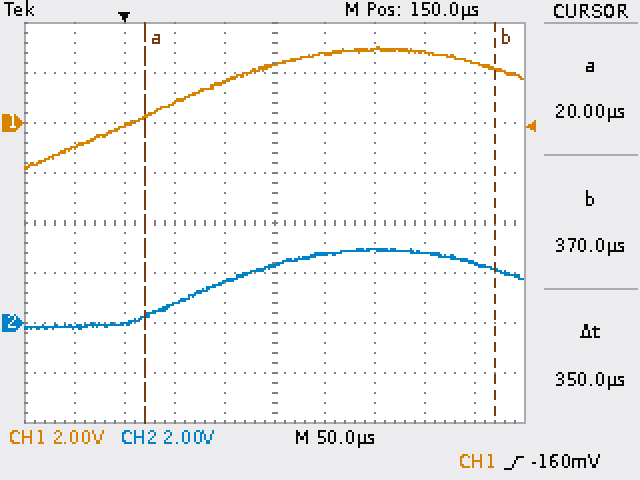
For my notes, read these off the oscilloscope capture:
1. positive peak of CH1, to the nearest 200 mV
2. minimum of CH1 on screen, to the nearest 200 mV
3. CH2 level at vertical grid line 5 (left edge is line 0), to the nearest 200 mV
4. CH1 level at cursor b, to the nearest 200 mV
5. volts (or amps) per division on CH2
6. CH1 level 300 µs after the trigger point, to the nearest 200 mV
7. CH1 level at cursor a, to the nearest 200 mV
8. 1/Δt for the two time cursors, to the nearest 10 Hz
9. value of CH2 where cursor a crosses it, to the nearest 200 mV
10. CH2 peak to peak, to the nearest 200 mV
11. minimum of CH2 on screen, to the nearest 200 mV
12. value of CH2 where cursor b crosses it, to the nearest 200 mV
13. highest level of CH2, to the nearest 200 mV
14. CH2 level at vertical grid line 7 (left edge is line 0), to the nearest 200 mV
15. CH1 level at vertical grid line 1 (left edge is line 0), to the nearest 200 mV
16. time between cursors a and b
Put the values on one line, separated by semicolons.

3.0 V; -1.8 V; 2.4 V; 2.2 V; 2 V; 2.8 V; 200 mV; 2.86 kHz; 200 mV; 3.2 V; -200 mV; 2.2 V; 3.0 V; 3.0 V; -1.0 V; 350 µs
